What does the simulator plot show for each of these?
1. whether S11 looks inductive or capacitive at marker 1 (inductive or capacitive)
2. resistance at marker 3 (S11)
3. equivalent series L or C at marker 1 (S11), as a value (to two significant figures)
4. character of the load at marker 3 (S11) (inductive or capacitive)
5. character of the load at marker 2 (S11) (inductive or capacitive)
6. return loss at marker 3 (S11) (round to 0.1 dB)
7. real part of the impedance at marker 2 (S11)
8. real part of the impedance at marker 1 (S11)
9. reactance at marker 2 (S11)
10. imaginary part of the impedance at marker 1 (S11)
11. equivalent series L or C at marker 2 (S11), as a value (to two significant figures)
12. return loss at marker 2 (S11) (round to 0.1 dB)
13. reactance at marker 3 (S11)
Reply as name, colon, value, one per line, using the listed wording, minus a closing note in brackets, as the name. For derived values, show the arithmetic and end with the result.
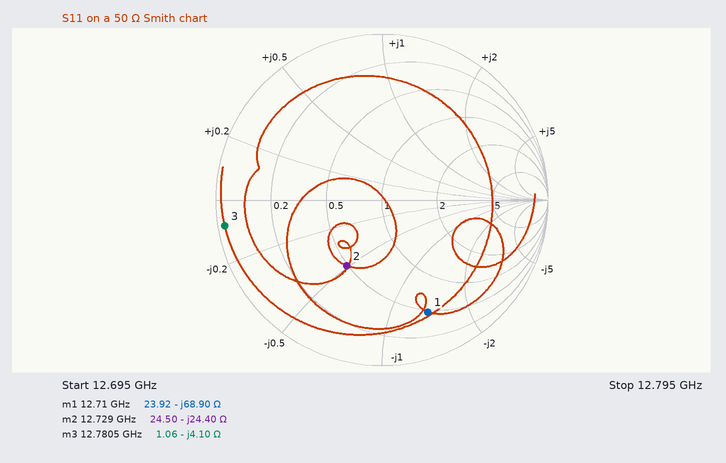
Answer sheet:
whether S11 looks inductive or capacitive at marker 1: capacitive
resistance at marker 3: 1.06 Ω
equivalent series L or C at marker 1 (S11), as a value: C = 1/(2π × 12.71 GHz × 68.9 Ω) ≈ 182 fF, so 180 fF to two significant figures
character of the load at marker 3 (S11): capacitive
character of the load at marker 2 (S11): capacitive
return loss at marker 3 (S11): 0.4 dB
real part of the impedance at marker 2: 24.50 Ω
real part of the impedance at marker 1: 23.92 Ω
reactance at marker 2: -24.40 Ω
imaginary part of the impedance at marker 1: -68.90 Ω
equivalent series L or C at marker 2 (S11), as a value: C = 1/(2π × 12.729 GHz × 24.4 Ω) ≈ 512 fF, so 510 fF to two significant figures
return loss at marker 2 (S11): 6.9 dB
reactance at marker 3: -4.10 Ω
